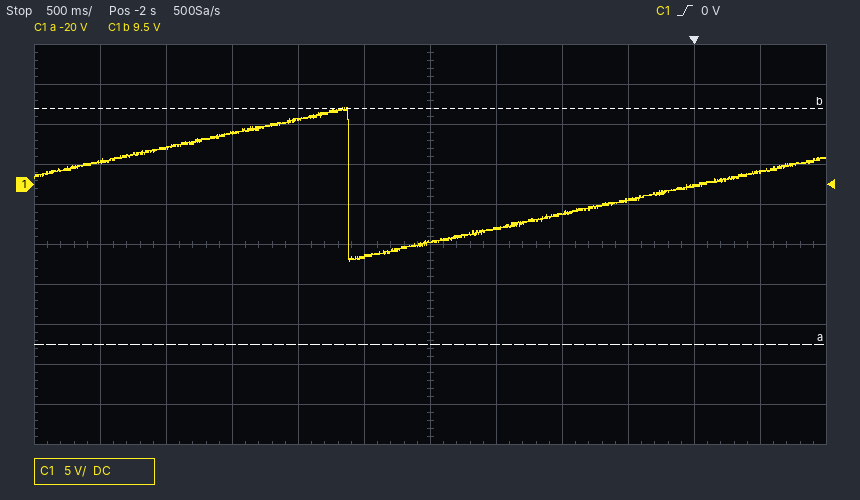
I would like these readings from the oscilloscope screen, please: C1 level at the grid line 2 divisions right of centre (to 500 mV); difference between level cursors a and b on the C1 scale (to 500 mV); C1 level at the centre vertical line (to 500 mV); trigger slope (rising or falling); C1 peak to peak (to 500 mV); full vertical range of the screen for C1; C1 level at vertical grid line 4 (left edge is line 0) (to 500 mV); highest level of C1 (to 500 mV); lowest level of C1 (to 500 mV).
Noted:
-3.5 V
29.5 V
-7.0 V
rising
19.0 V
50 V
8.0 V
9.5 V
-9.5 V
